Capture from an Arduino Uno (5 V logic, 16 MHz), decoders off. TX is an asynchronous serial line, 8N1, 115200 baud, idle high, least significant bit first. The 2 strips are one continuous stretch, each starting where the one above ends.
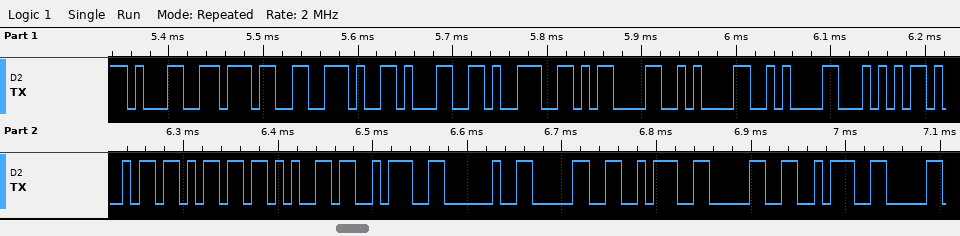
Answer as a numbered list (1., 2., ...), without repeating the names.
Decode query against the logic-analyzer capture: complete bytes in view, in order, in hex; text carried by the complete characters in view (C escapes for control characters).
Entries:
1. 31 37 2E 31 39 0D 0A 0A 54 69 6D 65 3A 20 30 3A 30 3A
2. "17.19\r\n\nTime: 0:0:"
